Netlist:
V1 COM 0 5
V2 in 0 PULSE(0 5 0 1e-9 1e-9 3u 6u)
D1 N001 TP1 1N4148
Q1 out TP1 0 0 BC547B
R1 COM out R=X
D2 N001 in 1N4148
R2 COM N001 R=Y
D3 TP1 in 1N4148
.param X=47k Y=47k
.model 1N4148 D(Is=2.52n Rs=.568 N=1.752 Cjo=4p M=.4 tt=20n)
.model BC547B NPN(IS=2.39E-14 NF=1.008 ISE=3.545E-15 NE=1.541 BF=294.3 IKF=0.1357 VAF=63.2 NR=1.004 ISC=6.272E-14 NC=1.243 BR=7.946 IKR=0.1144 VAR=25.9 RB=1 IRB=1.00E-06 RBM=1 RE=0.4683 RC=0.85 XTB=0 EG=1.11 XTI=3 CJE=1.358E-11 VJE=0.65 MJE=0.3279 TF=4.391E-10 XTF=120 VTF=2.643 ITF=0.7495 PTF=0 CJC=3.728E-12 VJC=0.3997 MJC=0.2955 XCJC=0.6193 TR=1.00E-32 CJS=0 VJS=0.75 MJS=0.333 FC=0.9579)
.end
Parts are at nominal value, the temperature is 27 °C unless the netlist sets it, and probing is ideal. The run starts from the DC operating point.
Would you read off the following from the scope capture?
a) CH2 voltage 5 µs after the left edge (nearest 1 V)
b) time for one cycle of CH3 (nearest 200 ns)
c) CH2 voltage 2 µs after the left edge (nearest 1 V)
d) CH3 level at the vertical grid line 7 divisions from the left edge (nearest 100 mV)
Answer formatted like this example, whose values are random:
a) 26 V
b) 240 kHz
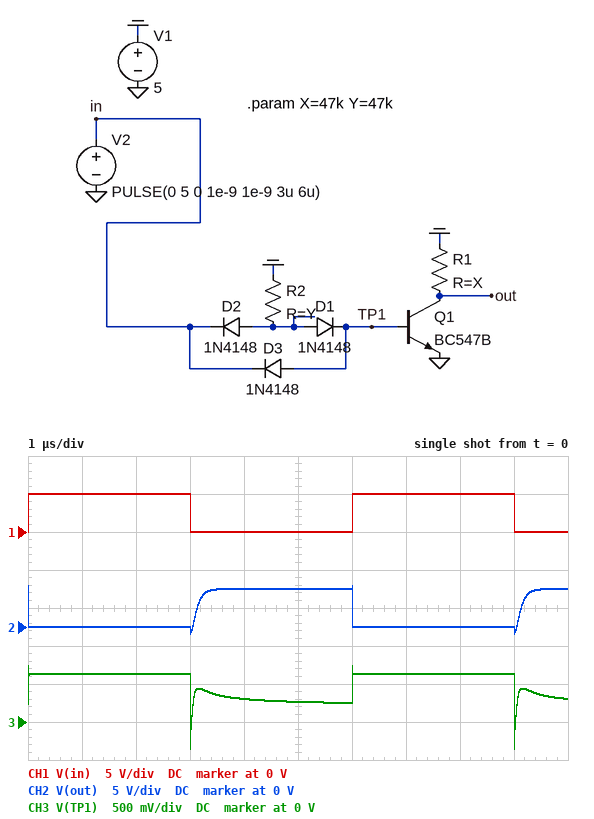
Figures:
a) 5 V
b) 6.0 µs
c) 0 V
d) 600 mV
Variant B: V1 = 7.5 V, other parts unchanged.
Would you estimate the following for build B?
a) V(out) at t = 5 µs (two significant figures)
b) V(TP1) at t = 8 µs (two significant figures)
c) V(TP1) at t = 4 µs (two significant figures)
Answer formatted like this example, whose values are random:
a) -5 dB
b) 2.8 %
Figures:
a) 7.5 V
b) 640 mV
c) 300 mV
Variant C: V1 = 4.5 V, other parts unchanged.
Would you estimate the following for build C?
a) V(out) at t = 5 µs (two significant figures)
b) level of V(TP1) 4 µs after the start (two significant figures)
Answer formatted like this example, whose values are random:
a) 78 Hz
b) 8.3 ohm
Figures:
a) 4.5 V
b) 300 mV
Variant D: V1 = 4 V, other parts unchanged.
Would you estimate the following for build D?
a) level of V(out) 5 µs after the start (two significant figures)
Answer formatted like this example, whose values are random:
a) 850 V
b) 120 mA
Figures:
a) 4.0 V
